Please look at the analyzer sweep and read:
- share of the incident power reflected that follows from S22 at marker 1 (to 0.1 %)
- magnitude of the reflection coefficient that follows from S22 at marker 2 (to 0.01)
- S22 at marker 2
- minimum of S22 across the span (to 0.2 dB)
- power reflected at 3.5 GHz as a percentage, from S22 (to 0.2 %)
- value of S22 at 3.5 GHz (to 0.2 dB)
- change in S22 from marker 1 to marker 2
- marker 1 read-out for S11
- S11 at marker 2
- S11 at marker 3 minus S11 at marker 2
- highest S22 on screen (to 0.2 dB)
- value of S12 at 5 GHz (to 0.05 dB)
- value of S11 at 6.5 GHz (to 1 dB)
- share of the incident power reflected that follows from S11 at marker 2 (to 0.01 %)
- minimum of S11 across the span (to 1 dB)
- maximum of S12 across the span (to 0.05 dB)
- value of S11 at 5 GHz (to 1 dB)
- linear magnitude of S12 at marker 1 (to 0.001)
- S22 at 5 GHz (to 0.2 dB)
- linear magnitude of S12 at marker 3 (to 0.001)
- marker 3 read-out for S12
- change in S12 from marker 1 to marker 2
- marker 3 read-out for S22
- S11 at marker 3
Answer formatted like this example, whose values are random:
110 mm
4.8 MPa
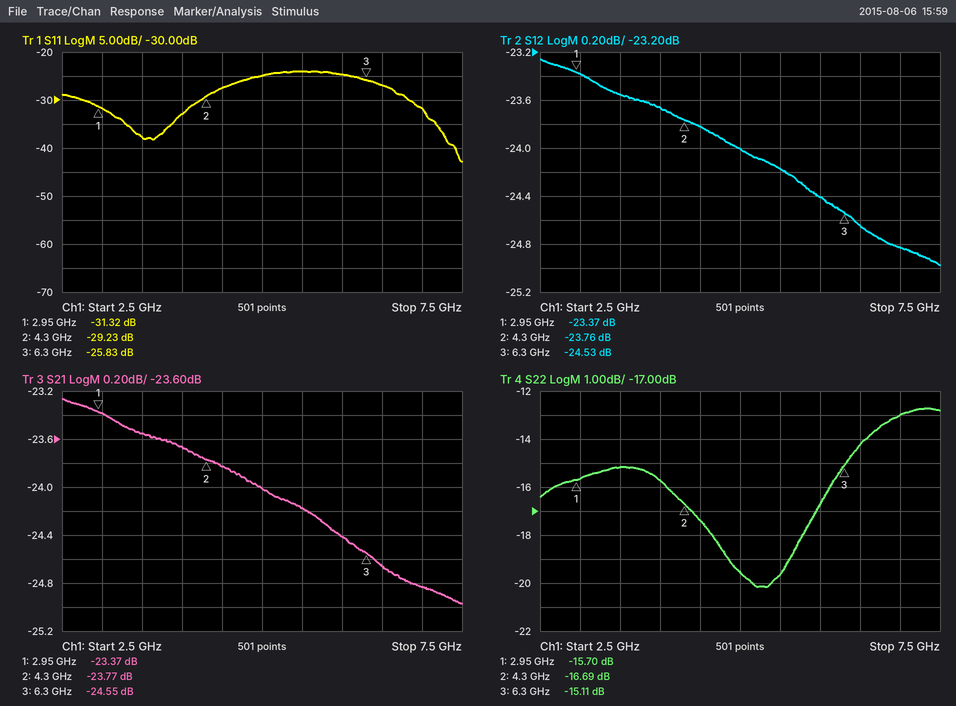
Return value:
2.7 %
0.15
-16.69 dB
-20.2 dB
3.0 %
-15.2 dB
-0.99 dB
-31.32 dB
-29.23 dB
3.40 dB
-12.8 dB
-24.00 dB
-27 dB
0.12 %
-43 dB
-23.25 dB
-25 dB
0.068
-19.6 dB
0.059
-24.53 dB
-0.39 dB
-15.11 dB
-25.83 dB
